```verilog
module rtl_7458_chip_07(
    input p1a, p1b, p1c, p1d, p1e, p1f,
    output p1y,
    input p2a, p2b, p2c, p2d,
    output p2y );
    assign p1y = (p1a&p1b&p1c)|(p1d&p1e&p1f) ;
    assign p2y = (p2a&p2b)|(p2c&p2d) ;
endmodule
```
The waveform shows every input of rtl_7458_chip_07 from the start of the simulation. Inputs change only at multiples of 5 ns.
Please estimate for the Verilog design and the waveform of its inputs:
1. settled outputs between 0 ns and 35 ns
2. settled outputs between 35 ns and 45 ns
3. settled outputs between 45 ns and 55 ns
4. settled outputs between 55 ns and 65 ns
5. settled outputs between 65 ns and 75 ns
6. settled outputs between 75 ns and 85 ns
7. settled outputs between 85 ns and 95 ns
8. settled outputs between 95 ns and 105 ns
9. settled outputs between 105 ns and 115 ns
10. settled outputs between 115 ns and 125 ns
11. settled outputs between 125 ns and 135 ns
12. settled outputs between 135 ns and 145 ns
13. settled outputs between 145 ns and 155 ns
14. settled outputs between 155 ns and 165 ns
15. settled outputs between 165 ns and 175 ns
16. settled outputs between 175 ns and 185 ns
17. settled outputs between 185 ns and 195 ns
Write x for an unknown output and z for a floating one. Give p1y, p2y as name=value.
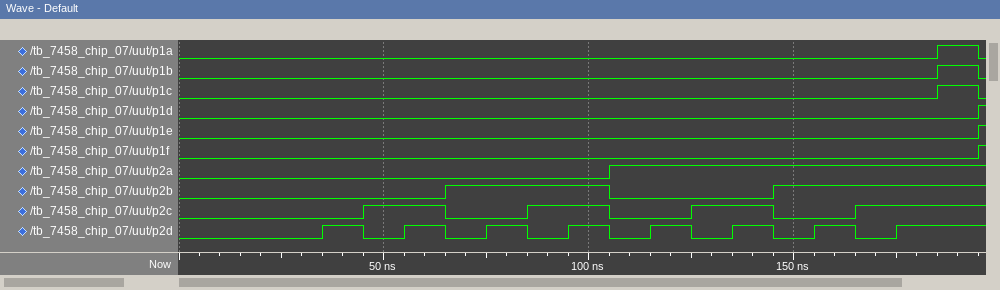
p1y=0, p2y=0
p1y=0, p2y=0
p1y=0, p2y=0
p1y=0, p2y=1
p1y=0, p2y=0
p1y=0, p2y=0
p1y=0, p2y=0
p1y=0, p2y=1
p1y=0, p2y=0
p1y=0, p2y=0
p1y=0, p2y=0
p1y=0, p2y=1
p1y=0, p2y=1
p1y=0, p2y=1
p1y=0, p2y=1
p1y=0, p2y=1
p1y=1, p2y=1
